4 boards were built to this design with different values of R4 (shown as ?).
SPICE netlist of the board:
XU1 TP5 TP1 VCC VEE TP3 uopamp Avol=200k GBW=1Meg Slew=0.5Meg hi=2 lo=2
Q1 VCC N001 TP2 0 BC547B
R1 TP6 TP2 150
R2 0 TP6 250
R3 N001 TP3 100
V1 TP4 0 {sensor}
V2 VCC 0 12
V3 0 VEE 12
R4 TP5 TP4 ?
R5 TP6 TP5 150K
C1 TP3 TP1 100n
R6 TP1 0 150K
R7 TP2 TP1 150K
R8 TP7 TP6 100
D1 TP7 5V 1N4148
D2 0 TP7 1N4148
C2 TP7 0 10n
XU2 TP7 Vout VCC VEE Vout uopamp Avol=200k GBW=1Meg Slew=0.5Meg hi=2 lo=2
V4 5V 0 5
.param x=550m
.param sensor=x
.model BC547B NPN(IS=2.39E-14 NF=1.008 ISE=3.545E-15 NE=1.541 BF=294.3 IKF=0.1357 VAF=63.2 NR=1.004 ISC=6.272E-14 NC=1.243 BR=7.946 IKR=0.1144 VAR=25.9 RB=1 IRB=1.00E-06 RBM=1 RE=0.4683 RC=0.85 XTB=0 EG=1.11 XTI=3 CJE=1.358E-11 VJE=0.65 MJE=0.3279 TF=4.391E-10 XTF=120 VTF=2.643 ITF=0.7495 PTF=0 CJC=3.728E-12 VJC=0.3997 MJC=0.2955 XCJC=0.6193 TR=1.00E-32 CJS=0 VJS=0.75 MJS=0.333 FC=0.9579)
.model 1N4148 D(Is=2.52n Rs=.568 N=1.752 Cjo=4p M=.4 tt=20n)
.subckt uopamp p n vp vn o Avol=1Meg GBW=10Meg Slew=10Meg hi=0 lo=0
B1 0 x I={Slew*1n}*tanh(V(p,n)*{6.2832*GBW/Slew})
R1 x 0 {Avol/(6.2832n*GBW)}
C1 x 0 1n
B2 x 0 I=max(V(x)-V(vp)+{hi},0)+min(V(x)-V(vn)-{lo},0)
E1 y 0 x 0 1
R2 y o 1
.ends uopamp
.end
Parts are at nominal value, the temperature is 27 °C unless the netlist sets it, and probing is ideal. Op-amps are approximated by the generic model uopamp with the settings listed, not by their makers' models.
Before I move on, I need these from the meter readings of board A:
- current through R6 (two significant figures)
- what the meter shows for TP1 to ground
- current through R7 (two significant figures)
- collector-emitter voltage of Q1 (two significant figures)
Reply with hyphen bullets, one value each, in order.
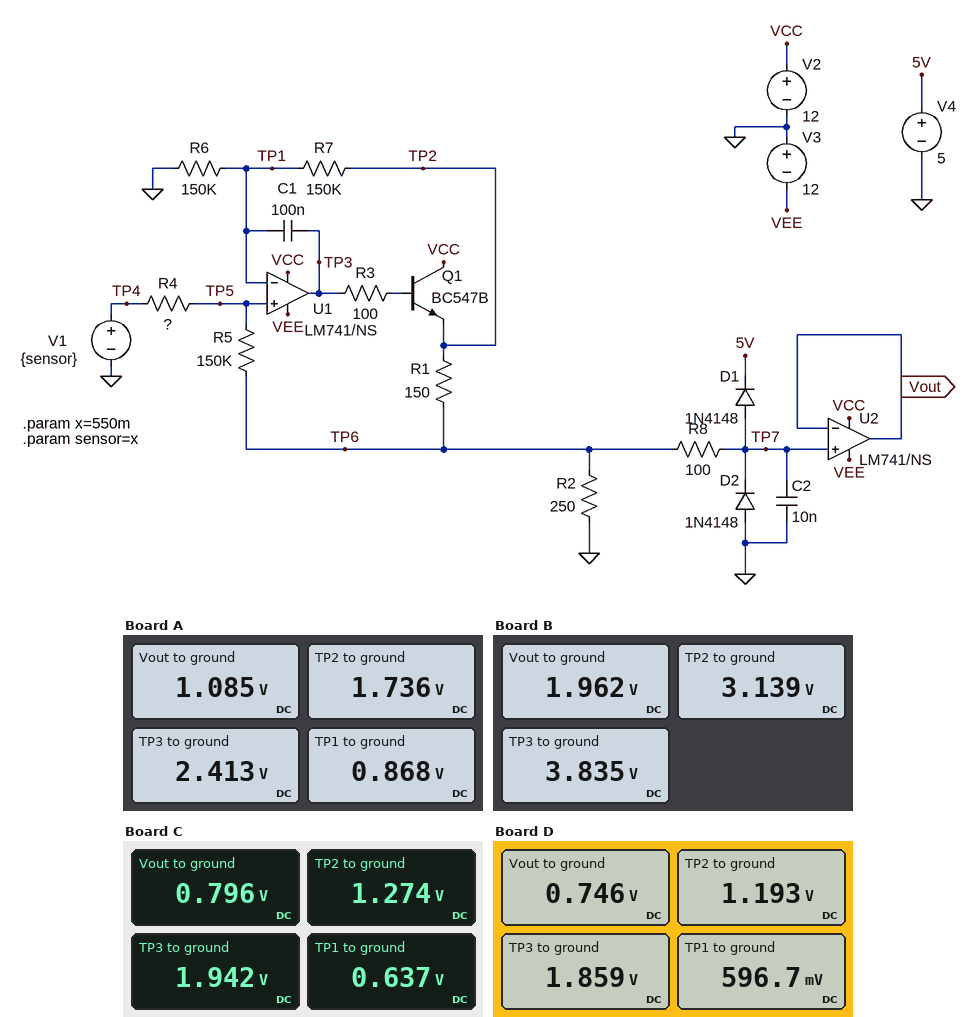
- 5.8 µA
- 0.868 V
- 5.8 µA
- 10 V
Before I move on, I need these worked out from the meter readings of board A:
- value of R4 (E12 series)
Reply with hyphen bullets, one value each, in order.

- 220 kΩ
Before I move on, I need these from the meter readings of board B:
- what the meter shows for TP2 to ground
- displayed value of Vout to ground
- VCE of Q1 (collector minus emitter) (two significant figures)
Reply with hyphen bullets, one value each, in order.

- 3.139 V
- 1.962 V
- 8.9 V
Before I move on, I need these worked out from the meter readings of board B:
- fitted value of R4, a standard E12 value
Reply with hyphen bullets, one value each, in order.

- 390 kΩ
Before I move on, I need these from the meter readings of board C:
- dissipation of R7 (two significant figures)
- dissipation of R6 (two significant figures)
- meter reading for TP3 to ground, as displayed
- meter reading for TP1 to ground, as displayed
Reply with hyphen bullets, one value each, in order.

- 2.7 µW
- 2.7 µW
- 1.942 V
- 0.637 V
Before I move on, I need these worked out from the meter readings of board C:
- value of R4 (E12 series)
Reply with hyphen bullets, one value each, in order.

- 82 kΩ
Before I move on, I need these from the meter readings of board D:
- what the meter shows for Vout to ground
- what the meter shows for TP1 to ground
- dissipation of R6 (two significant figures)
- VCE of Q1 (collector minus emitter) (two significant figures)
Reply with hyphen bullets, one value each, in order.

- 0.746 V
- 596.7 mV
- 2.4 µW
- 11 V
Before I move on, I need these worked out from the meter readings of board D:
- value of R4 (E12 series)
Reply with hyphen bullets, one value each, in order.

- 47 kΩ
